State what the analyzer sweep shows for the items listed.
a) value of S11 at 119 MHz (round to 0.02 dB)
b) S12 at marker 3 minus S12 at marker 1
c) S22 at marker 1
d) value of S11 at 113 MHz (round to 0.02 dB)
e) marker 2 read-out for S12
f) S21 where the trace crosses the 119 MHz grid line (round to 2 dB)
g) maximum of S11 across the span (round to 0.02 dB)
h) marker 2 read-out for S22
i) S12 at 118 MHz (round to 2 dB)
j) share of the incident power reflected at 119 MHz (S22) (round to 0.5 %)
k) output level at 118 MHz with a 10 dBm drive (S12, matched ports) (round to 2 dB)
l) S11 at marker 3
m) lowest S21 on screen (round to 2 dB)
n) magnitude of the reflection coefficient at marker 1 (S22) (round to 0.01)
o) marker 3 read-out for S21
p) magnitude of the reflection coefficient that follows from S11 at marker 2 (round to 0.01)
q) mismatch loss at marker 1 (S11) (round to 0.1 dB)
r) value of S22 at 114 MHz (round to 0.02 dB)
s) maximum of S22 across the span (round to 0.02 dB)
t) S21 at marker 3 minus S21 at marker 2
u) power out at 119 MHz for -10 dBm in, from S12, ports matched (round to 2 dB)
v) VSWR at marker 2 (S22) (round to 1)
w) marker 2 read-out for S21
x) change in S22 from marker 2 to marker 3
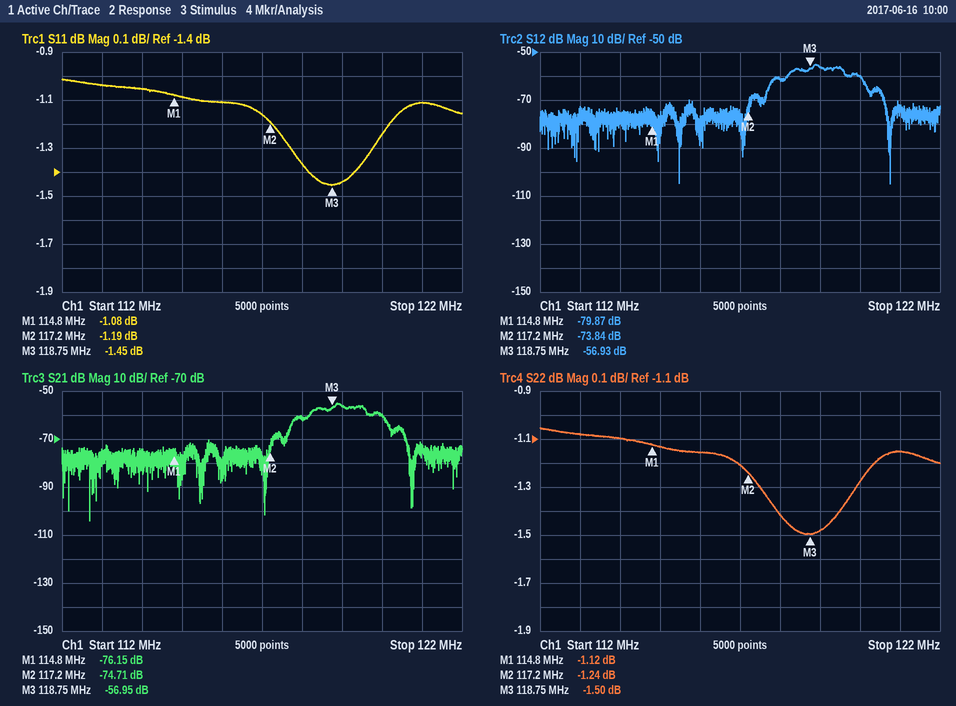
-1.44 dB
22.94 dB
-1.12 dB
-1.04 dB
-73.84 dB
-56 dB
-1.02 dB
-1.24 dB
-62 dB
71.0 %
-52 dBm
-1.45 dB
-104 dB
0.88
-56.95 dB
0.87
6.6 dB
-1.10 dB
-1.06 dB
17.76 dB
-66 dBm
14
-74.71 dB
-0.26 dB
